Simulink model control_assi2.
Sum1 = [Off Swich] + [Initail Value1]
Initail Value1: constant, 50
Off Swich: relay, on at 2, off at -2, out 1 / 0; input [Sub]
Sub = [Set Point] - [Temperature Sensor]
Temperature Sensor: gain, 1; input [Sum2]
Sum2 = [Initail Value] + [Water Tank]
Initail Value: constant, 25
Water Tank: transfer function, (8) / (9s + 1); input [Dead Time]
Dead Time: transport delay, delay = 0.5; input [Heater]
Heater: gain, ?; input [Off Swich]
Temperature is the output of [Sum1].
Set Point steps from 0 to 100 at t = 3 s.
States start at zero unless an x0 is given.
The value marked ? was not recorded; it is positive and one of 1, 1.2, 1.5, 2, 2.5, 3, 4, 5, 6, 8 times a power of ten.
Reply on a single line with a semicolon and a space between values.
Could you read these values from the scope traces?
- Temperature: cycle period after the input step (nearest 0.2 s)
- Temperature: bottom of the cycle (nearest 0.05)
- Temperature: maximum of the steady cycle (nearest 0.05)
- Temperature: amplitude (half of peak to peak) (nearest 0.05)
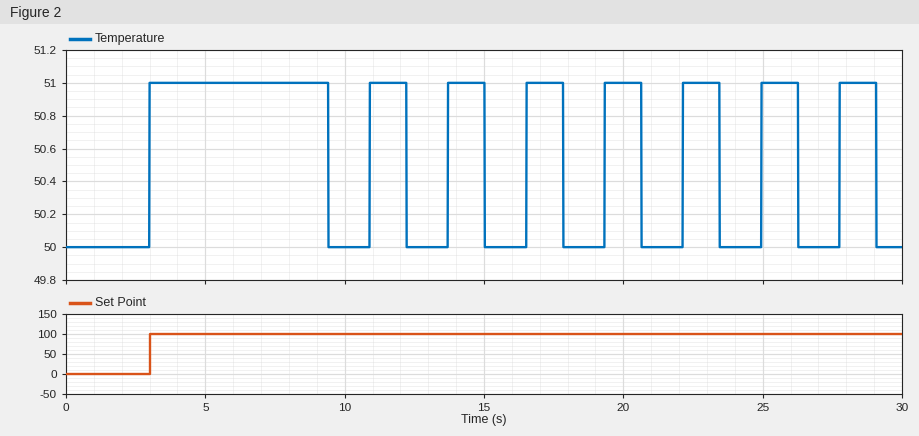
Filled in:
2.8 s; 50.00; 51.00; 0.50
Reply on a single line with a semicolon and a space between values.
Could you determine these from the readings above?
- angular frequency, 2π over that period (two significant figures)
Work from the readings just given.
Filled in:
2.2 rad/s
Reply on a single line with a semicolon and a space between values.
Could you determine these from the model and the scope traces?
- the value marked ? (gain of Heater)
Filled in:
20
